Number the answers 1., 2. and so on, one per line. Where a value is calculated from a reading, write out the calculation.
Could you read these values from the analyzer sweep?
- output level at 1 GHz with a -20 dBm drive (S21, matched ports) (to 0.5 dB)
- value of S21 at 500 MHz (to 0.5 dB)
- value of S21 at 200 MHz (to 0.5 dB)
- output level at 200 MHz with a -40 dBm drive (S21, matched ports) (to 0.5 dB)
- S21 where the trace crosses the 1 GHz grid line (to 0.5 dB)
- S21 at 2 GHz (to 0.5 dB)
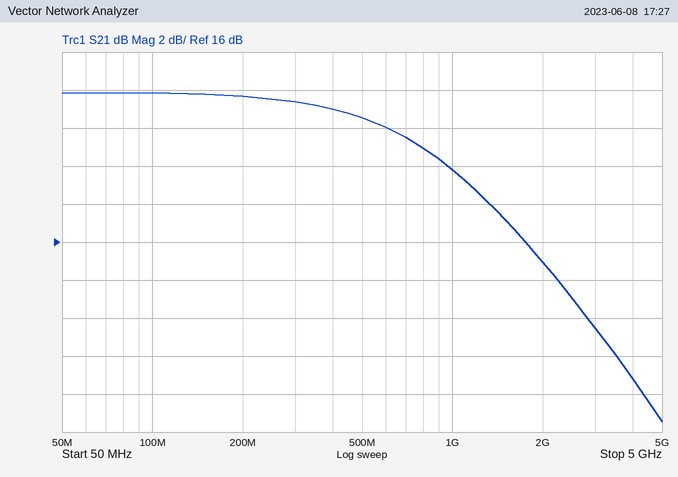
1. -20 dBm + (20.0 dB) = 0.0 dBm
2. 22.5 dB
3. 23.5 dB
4. -40 dBm + (23.5 dB) = -16.5 dBm
5. 20.0 dB
6. 15.0 dB
